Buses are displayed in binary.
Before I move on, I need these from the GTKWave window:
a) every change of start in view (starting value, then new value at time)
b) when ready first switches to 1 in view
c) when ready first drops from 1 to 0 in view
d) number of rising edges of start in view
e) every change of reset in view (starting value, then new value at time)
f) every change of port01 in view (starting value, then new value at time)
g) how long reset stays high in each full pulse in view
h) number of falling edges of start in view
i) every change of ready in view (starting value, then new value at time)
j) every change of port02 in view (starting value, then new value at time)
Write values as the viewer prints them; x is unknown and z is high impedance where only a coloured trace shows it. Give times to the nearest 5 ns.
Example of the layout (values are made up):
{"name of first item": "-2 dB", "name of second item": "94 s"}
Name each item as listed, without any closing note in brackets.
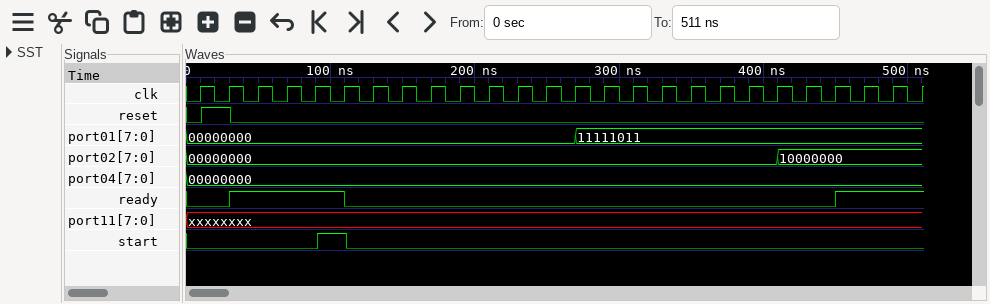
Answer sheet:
{"every change of start in view": "0, 1 at 90 ns, 0 at 110 ns", "when ready first switches to 1 in view": "30 ns", "when ready first drops from 1 to 0 in view": "110 ns", "number of rising edges of start in view": "1", "every change of reset in view": "0, 1 at 10 ns, 0 at 30 ns", "every change of port01 in view": "00000000, 11111011 at 270 ns", "how long reset stays high in each full pulse in view": "20 ns", "number of falling edges of start in view": "1", "every change of ready in view": "0, 1 at 30 ns, 0 at 110 ns, 1 at 450 ns", "every change of port02 in view": "00000000, 10000000 at 410 ns"}
